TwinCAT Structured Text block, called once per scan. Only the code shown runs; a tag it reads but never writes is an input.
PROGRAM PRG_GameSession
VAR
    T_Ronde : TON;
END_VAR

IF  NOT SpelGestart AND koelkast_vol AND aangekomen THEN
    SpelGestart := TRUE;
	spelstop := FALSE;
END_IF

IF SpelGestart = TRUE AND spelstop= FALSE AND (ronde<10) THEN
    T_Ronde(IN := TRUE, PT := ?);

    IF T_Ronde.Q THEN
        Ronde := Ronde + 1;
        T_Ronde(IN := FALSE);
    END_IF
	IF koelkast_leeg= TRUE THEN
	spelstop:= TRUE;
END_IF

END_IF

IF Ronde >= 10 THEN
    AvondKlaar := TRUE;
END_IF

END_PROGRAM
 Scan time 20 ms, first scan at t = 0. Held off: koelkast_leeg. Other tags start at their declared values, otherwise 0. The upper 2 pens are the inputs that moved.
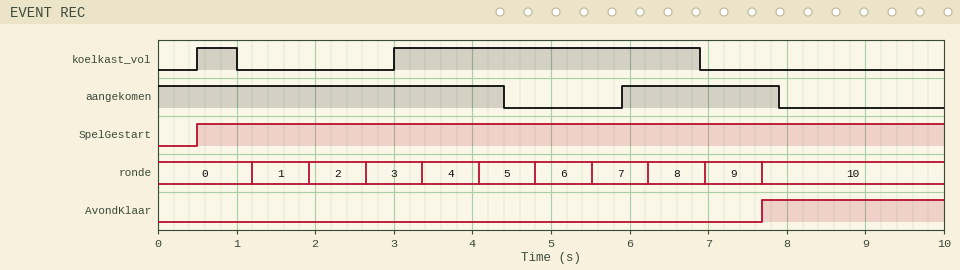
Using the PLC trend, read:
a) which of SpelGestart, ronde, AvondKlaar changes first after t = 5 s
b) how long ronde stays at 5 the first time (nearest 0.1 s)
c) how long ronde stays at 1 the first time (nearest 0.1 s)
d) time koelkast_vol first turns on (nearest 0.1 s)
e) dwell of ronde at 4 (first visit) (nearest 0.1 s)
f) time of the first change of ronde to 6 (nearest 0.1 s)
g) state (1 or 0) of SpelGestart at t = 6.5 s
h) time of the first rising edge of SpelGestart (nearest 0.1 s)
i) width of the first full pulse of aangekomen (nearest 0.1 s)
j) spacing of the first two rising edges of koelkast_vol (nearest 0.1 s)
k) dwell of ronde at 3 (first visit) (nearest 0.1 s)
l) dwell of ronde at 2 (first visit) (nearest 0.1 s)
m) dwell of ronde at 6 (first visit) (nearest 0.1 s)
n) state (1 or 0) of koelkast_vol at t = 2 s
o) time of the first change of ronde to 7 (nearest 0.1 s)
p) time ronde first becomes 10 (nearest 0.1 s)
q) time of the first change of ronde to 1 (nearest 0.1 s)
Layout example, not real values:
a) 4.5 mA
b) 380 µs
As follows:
a) ronde
b) 0.7 s
c) 0.7 s
d) 0.5 s
e) 0.7 s
f) 4.8 s
g) 1
h) 0.5 s
i) 2.0 s
j) 2.5 s
k) 0.7 s
l) 0.7 s
m) 0.7 s
n) 0
o) 5.5 s
p) 7.7 s
q) 1.2 s
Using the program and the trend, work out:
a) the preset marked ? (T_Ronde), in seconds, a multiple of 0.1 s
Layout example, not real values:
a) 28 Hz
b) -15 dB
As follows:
a) 0.7 s
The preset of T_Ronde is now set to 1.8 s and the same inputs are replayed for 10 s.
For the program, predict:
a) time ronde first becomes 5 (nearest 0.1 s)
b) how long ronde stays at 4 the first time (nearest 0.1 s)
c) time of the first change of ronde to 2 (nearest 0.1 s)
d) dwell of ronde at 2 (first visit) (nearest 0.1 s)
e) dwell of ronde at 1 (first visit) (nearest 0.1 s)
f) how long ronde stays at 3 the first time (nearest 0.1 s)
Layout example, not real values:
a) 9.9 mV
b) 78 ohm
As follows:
a) 9.6 s
b) 1.8 s
c) 4.1 s
d) 1.8 s
e) 1.8 s
f) 1.8 s
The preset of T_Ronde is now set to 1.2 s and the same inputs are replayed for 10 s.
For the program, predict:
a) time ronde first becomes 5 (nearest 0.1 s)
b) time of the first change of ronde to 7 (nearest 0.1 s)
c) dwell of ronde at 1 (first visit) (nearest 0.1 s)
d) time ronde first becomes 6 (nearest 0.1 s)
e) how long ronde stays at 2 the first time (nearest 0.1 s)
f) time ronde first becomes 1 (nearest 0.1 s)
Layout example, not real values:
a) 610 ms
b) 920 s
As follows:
a) 6.6 s
b) 9.0 s
c) 1.2 s
d) 7.8 s
e) 1.2 s
f) 1.7 s
